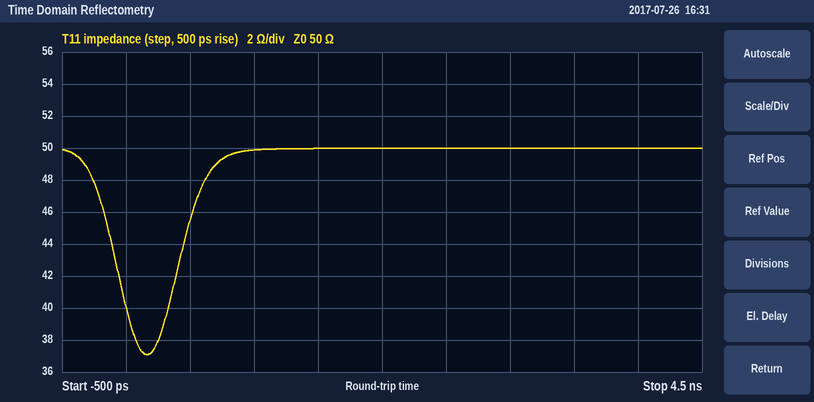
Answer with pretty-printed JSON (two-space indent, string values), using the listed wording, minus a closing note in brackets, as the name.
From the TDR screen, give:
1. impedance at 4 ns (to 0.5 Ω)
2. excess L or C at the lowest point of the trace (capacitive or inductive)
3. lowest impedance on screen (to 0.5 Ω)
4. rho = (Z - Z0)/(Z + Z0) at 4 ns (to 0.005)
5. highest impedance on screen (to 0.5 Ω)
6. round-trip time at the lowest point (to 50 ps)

{
  "impedance at 4 ns": "50.0 Ω",
  "excess L or C at the lowest point of the trace": "capacitive",
  "lowest impedance on screen": "37.0 Ω",
  "rho = (Z - Z0)/(Z + Z0) at 4 ns": "0.000",
  "highest impedance on screen": "50.0 Ω",
  "round-trip time at the lowest point": "150 ps"
}
